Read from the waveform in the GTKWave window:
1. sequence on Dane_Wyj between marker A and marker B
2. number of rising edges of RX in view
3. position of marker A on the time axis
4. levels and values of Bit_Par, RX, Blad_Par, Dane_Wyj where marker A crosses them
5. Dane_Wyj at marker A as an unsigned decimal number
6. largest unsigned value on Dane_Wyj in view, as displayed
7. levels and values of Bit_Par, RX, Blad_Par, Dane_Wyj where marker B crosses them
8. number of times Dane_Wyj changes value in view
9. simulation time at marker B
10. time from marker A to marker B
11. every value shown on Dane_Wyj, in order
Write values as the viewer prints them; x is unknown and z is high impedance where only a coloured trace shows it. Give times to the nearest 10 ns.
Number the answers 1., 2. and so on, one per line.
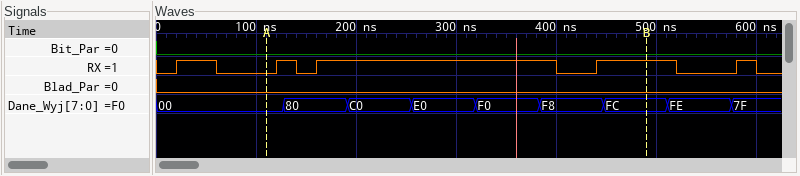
1. 00, 80, C0, E0, F0, F8, FC
2. 5
3. 110 ns
4. Bit_Par=0, RX=0, Blad_Par=0, Dane_Wyj=00
5. 0
6. FE
7. Bit_Par=0, RX=1, Blad_Par=0, Dane_Wyj=FC
8. 8
9. 490 ns
10. 380 ns
11. 00, 80, C0, E0, F0, F8, FC, FE, 7F
